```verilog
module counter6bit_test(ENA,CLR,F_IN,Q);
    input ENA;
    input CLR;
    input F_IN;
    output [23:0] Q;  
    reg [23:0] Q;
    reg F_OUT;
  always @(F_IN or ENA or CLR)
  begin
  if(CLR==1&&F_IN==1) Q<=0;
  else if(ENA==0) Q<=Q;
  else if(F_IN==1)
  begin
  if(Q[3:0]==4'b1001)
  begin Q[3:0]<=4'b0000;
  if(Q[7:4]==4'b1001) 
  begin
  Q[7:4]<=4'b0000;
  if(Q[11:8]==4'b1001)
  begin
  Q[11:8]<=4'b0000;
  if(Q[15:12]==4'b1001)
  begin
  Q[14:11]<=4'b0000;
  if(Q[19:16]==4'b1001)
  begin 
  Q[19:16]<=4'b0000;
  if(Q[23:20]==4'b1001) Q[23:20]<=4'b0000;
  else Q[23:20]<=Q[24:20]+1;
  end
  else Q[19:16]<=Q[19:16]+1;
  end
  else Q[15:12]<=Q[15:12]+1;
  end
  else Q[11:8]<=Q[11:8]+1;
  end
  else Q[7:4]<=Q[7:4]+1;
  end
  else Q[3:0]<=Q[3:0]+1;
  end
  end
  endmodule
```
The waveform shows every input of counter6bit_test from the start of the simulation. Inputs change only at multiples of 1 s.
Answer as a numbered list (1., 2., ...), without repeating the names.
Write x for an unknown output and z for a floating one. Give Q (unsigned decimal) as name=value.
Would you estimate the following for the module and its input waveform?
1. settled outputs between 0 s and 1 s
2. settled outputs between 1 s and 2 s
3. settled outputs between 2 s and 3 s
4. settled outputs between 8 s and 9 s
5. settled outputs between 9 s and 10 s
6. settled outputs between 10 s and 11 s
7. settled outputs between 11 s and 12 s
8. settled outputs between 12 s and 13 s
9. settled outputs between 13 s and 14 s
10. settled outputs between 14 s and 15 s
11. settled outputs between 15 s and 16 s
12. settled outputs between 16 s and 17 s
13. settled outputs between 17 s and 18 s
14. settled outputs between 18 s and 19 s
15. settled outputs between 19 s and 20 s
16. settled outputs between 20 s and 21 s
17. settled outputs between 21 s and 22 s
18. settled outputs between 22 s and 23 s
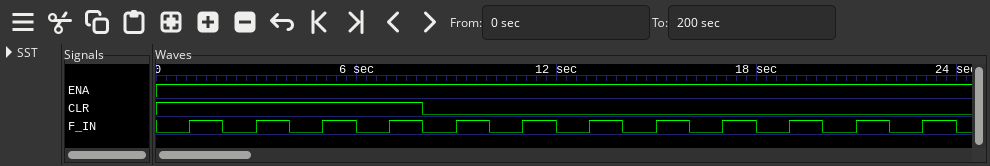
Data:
1. Q=x
2. Q=0
3. Q=0
4. Q=0
5. Q=1
6. Q=1
7. Q=2
8. Q=2
9. Q=3
10. Q=3
11. Q=4
12. Q=4
13. Q=5
14. Q=5
15. Q=6
16. Q=6
17. Q=7
18. Q=7
